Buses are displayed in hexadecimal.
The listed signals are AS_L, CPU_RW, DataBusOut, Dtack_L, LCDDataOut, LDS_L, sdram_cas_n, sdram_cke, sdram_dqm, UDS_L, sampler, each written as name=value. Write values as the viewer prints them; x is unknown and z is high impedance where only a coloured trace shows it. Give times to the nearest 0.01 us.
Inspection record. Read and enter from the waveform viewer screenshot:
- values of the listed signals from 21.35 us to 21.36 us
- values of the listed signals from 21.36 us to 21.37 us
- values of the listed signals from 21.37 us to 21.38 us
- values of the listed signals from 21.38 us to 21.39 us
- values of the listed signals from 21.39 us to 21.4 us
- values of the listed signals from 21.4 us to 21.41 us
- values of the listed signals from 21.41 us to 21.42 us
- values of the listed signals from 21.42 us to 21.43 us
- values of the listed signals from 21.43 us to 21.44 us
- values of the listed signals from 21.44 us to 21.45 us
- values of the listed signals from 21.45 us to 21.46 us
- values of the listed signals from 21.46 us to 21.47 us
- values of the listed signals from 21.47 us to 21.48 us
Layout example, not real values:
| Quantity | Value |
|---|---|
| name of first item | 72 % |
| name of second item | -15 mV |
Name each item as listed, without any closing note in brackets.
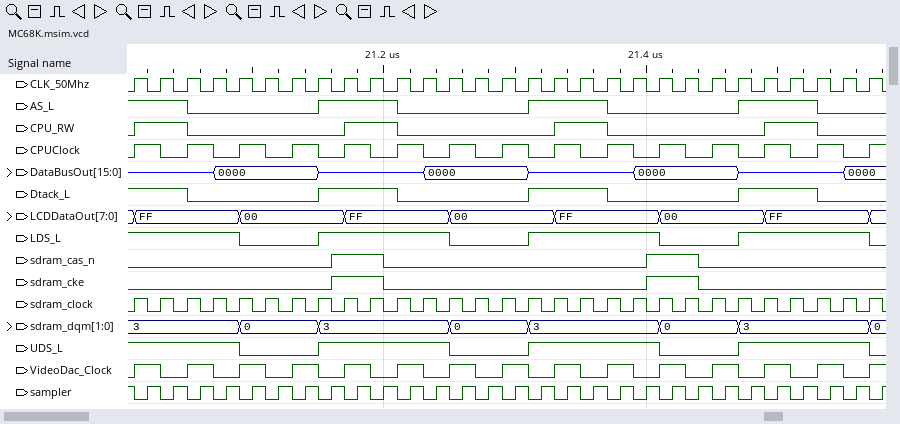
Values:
| Quantity | Value |
|---|---|
| values of the listed signals from 21.35 us to 21.36 us | AS_L=1, CPU_RW=1, DataBusOut=z, Dtack_L=1, LCDDataOut=FF, LDS_L=1, sdram_cas_n=0, sdram_cke=0, sdram_dqm=3, UDS_L=1, sampler=0 |
| values of the listed signals from 21.36 us to 21.37 us | AS_L=1, CPU_RW=1, DataBusOut=z, Dtack_L=1, LCDDataOut=FF, LDS_L=1, sdram_cas_n=0, sdram_cke=0, sdram_dqm=3, UDS_L=1, sampler=1 |
| values of the listed signals from 21.37 us to 21.38 us | AS_L=0, CPU_RW=0, DataBusOut=z, Dtack_L=0, LCDDataOut=FF, LDS_L=1, sdram_cas_n=0, sdram_cke=0, sdram_dqm=3, UDS_L=1, sampler=0 |
| values of the listed signals from 21.38 us to 21.39 us | AS_L=0, CPU_RW=0, DataBusOut=z, Dtack_L=0, LCDDataOut=FF, LDS_L=1, sdram_cas_n=0, sdram_cke=0, sdram_dqm=3, UDS_L=1, sampler=1 |
| values of the listed signals from 21.39 us to 21.4 us | AS_L=0, CPU_RW=0, DataBusOut=0000, Dtack_L=0, LCDDataOut=FF, LDS_L=1, sdram_cas_n=0, sdram_cke=0, sdram_dqm=3, UDS_L=1, sampler=0 |
| values of the listed signals from 21.4 us to 21.41 us | AS_L=0, CPU_RW=0, DataBusOut=0000, Dtack_L=0, LCDDataOut=FF, LDS_L=1, sdram_cas_n=1, sdram_cke=1, sdram_dqm=3, UDS_L=1, sampler=1 |
| values of the listed signals from 21.41 us to 21.42 us | AS_L=0, CPU_RW=0, DataBusOut=0000, Dtack_L=0, LCDDataOut=00, LDS_L=0, sdram_cas_n=1, sdram_cke=1, sdram_dqm=0, UDS_L=0, sampler=0 |
| values of the listed signals from 21.42 us to 21.43 us | AS_L=0, CPU_RW=0, DataBusOut=0000, Dtack_L=0, LCDDataOut=00, LDS_L=0, sdram_cas_n=1, sdram_cke=1, sdram_dqm=0, UDS_L=0, sampler=1 |
| values of the listed signals from 21.43 us to 21.44 us | AS_L=0, CPU_RW=0, DataBusOut=0000, Dtack_L=0, LCDDataOut=00, LDS_L=0, sdram_cas_n=1, sdram_cke=1, sdram_dqm=0, UDS_L=0, sampler=0 |
| values of the listed signals from 21.44 us to 21.45 us | AS_L=0, CPU_RW=0, DataBusOut=0000, Dtack_L=0, LCDDataOut=00, LDS_L=0, sdram_cas_n=0, sdram_cke=0, sdram_dqm=0, UDS_L=0, sampler=1 |
| values of the listed signals from 21.45 us to 21.46 us | AS_L=0, CPU_RW=0, DataBusOut=0000, Dtack_L=0, LCDDataOut=00, LDS_L=0, sdram_cas_n=0, sdram_cke=0, sdram_dqm=0, UDS_L=0, sampler=0 |
| values of the listed signals from 21.46 us to 21.47 us | AS_L=0, CPU_RW=0, DataBusOut=0000, Dtack_L=0, LCDDataOut=00, LDS_L=0, sdram_cas_n=0, sdram_cke=0, sdram_dqm=0, UDS_L=0, sampler=1 |
| values of the listed signals from 21.47 us to 21.48 us | AS_L=1, CPU_RW=0, DataBusOut=z, Dtack_L=1, LCDDataOut=00, LDS_L=1, sdram_cas_n=0, sdram_cke=0, sdram_dqm=3, UDS_L=1, sampler=0 |
